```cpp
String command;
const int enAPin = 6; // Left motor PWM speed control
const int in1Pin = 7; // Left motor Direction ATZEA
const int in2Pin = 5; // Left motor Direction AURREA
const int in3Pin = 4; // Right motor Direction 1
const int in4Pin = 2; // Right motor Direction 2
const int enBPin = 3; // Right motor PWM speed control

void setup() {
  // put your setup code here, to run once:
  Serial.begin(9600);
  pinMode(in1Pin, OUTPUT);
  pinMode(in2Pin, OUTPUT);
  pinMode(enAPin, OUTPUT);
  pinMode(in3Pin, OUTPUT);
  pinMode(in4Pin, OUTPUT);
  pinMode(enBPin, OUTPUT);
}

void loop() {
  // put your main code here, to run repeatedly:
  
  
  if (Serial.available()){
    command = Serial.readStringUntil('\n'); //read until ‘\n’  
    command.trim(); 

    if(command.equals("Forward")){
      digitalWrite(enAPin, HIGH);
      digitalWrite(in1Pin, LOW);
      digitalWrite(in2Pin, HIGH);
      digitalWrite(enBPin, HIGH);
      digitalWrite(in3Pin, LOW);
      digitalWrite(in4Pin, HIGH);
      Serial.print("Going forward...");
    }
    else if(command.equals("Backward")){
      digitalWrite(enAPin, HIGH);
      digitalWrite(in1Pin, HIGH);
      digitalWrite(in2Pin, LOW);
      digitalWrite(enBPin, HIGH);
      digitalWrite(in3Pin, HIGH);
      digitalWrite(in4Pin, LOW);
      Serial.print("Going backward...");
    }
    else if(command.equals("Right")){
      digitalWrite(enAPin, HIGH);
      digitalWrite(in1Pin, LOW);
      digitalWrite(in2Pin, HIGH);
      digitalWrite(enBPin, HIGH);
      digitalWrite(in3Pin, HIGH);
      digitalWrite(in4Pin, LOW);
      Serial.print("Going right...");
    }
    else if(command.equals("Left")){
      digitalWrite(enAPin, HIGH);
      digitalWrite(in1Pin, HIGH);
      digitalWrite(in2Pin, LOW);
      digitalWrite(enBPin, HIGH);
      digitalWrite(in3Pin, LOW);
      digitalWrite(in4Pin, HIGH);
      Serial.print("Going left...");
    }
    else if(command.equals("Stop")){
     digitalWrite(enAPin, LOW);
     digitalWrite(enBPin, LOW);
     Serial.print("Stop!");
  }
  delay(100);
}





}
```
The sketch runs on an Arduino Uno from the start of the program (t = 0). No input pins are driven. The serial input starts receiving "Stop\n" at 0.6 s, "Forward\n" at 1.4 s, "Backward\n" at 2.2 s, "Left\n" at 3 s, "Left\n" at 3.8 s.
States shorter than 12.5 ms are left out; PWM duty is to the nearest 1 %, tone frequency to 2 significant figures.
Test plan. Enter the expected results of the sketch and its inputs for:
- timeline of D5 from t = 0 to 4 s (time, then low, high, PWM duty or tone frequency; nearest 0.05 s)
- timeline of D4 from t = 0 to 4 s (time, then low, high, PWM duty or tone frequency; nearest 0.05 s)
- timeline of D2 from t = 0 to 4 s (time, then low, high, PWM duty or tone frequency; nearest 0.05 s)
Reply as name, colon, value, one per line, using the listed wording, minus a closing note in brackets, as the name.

timeline of D5 from t = 0 to 4 s: 0 s low; 1.4 s high; 2.2 s low
timeline of D4 from t = 0 to 4 s: 0 s low; 2.2 s high; 3 s low
timeline of D2 from t = 0 to 4 s: 0 s low; 1.4 s high; 2.2 s low; 3 s high
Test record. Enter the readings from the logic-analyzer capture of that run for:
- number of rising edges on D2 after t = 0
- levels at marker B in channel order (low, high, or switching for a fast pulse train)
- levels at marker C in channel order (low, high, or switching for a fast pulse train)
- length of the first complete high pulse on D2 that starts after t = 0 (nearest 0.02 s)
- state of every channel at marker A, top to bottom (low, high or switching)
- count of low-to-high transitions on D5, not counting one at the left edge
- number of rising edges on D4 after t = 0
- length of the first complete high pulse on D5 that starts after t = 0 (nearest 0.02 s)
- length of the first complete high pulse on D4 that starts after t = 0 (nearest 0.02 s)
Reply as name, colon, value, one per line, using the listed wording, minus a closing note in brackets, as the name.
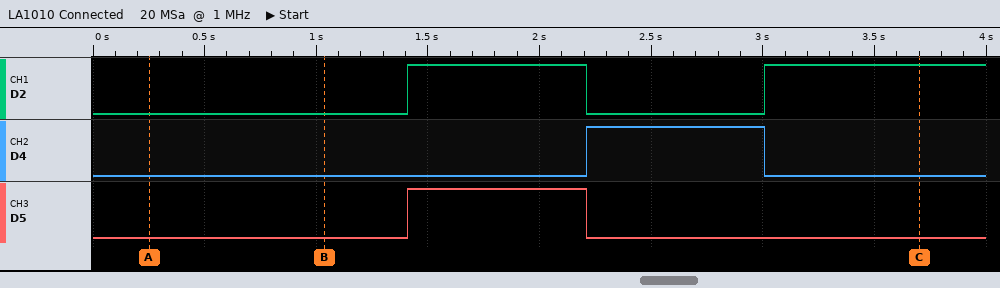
number of rising edges on D2 after t = 0: 2
levels at marker B in channel order: D2 low, D4 low, D5 low
levels at marker C in channel order: D2 high, D4 low, D5 low
length of the first complete high pulse on D2 that starts after t = 0: 0.80 s
state of every channel at marker A, top to bottom: D2 low, D4 low, D5 low
count of low-to-high transitions on D5, not counting one at the left edge: 1
number of rising edges on D4 after t = 0: 1
length of the first complete high pulse on D5 that starts after t = 0: 0.80 s
length of the first complete high pulse on D4 that starts after t = 0: 0.80 s
